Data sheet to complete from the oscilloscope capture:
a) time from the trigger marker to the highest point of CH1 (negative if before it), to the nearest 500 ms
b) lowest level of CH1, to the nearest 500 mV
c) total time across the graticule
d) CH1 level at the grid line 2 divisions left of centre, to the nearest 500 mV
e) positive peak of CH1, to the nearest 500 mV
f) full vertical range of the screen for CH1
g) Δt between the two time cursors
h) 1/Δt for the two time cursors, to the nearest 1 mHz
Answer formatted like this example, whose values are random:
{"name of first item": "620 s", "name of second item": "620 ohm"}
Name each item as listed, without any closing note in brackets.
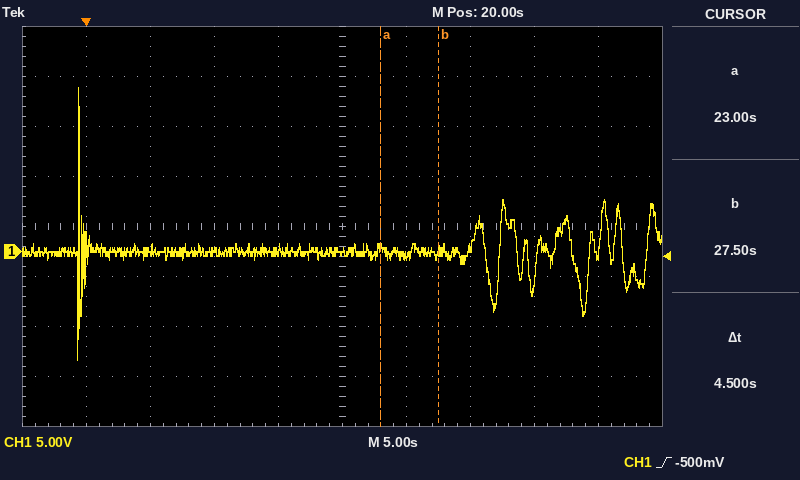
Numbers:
{"time from the trigger marker to the highest point of CH1 (negative if before it), to the nearest 500 ms": "-500 ms", "lowest level of CH1, to the nearest 500 mV": "-11.0 V", "total time across the graticule": "50 s", "CH1 level at the grid line 2 divisions left of centre, to the nearest 500 mV": "0.0 V", "positive peak of CH1, to the nearest 500 mV": "16.5 V", "full vertical range of the screen for CH1": "40 V", "Δt between the two time cursors": "4.5 s", "1/Δt for the two time cursors, to the nearest 1 mHz": "222 mHz"}
